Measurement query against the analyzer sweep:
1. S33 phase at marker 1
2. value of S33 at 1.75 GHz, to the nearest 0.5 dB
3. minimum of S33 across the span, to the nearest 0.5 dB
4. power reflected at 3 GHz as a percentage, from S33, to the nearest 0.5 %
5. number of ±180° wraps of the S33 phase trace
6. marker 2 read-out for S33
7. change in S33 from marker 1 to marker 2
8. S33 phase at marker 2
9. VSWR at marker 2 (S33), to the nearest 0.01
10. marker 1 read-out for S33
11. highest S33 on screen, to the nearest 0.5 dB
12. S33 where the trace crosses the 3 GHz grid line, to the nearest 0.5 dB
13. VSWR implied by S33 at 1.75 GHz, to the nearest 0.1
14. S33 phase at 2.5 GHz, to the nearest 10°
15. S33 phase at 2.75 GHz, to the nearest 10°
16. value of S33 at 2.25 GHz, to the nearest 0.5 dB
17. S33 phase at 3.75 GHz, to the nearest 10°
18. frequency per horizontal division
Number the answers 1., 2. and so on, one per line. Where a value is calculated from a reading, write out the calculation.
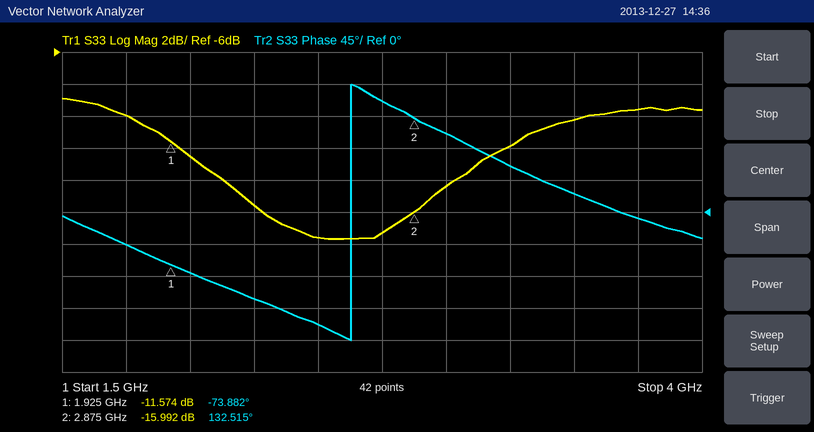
1. -73.882°
2. -10.0 dB
3. -17.5 dB
4. 10^(-14.5/10) ≈ 3.5 %
5. 1
6. -15.992 dB
7. -15.992 − (-11.574) = -4.418 dB
8. 132.515°
9. (1 + 0.1586)/(1 − 0.1586) ≈ 1.38
10. -11.574 dB
11. -9.0 dB
12. -14.5 dB
13. |Γ| = 10^(-10/20) = 0.3162; VSWR = (1 + 0.3162)/(1 − 0.3162) ≈ 1.9
14. -160°
15. 160°
16. -15.5 dB
17. -10°
18. 250 MHz
